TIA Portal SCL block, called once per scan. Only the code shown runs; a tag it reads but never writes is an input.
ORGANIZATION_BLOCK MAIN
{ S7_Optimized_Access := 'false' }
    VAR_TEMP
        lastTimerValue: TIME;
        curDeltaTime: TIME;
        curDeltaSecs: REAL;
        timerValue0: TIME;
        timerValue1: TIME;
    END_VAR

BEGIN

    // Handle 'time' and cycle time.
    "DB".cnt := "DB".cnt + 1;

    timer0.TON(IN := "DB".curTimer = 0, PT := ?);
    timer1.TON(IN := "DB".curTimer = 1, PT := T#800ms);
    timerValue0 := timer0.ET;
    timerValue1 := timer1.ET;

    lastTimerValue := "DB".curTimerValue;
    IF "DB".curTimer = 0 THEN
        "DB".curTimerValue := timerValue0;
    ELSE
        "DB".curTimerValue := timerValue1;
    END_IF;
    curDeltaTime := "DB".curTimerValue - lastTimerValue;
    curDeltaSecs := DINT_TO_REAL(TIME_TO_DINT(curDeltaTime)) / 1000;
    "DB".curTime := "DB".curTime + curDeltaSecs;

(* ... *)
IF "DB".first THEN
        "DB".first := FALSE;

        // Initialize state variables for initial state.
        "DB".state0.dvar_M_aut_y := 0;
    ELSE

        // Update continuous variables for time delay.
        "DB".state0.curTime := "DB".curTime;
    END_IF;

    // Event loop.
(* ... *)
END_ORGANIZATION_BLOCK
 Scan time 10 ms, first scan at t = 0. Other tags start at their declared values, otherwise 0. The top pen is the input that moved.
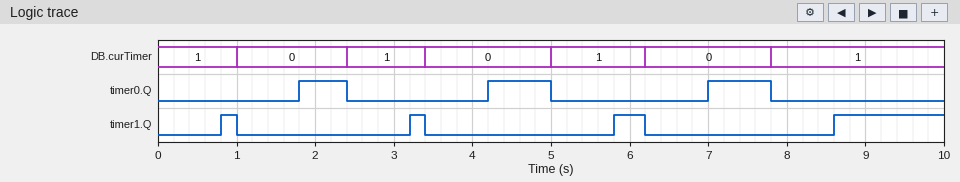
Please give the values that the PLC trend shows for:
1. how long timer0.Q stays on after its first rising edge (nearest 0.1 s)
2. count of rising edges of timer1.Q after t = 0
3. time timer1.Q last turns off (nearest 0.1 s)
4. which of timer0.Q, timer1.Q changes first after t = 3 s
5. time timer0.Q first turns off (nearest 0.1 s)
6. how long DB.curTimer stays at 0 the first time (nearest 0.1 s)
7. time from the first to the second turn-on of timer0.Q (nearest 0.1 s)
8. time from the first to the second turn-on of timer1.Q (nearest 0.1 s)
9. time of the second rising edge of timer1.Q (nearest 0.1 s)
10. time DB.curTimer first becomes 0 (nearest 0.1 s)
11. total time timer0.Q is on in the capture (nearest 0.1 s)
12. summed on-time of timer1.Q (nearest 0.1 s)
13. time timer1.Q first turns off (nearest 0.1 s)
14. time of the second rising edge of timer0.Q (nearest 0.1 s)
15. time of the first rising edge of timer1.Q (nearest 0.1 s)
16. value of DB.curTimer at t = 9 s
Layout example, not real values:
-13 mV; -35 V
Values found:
0.6 s; 4; 6.2 s; timer1.Q; 2.4 s; 1.4 s; 2.4 s; 2.4 s; 3.2 s; 1.0 s; 2.2 s; 2.2 s; 1.0 s; 4.2 s; 0.8 s; 1
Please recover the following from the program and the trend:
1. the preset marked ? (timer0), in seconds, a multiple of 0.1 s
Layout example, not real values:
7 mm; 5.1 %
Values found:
0.8 s
